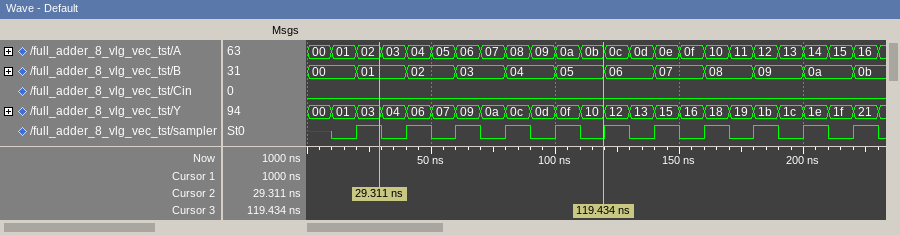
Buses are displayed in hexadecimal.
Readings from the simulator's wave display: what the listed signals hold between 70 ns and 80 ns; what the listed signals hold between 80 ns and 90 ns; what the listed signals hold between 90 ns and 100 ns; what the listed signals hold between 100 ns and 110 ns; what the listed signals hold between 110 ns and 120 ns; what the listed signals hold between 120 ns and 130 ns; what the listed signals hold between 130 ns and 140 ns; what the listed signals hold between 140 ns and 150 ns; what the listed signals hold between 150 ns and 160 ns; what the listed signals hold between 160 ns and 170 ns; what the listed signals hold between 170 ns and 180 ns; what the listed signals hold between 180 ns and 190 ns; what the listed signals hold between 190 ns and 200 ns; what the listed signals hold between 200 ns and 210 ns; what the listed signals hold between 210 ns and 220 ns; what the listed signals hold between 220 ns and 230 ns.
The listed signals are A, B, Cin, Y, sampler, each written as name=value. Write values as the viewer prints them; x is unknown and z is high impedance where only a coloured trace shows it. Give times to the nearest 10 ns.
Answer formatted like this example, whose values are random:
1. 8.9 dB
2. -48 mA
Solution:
1. A=07, B=03, Cin=0, Y=0a, sampler=0
2. A=08, B=04, Cin=0, Y=0c, sampler=1
3. A=09, B=04, Cin=0, Y=0d, sampler=0
4. A=0a, B=05, Cin=0, Y=0f, sampler=1
5. A=0b, B=05, Cin=0, Y=10, sampler=0
6. A=0c, B=06, Cin=0, Y=12, sampler=1
7. A=0d, B=06, Cin=0, Y=13, sampler=0
8. A=0e, B=07, Cin=0, Y=15, sampler=1
9. A=0f, B=07, Cin=0, Y=16, sampler=0
10. A=10, B=08, Cin=0, Y=18, sampler=1
11. A=11, B=08, Cin=0, Y=19, sampler=0
12. A=12, B=09, Cin=0, Y=1b, sampler=1
13. A=13, B=09, Cin=0, Y=1c, sampler=0
14. A=14, B=0a, Cin=0, Y=1e, sampler=1
15. A=15, B=0a, Cin=0, Y=1f, sampler=0
16. A=16, B=0b, Cin=0, Y=21, sampler=1
